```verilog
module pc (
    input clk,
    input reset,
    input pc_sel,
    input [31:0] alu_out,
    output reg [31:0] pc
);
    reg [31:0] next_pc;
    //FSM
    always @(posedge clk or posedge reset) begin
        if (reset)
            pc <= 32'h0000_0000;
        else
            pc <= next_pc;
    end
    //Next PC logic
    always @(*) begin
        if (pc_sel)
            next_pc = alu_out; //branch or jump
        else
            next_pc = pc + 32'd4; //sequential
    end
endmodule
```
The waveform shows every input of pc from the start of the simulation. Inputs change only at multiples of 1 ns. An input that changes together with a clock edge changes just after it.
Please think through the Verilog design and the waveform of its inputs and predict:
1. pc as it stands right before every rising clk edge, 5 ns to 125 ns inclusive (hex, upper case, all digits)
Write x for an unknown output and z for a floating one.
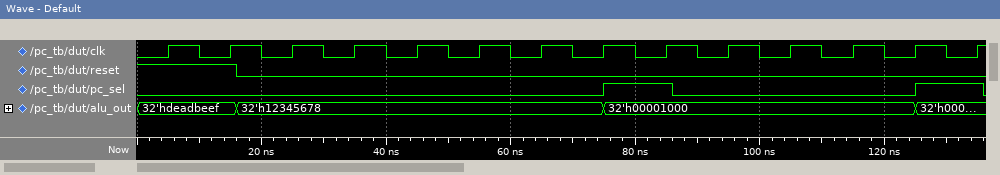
00000000, 00000000, 00000000, 00000004, 00000008, 0000000C, 00000010, 00000014, 00000018, 00001000, 00001004, 00001008, 0000100C
